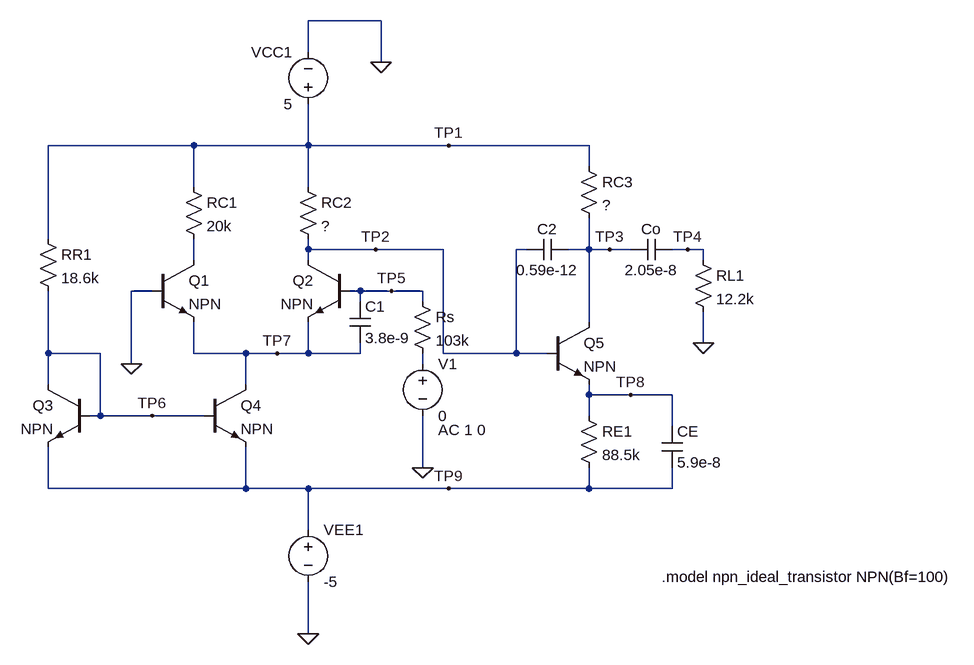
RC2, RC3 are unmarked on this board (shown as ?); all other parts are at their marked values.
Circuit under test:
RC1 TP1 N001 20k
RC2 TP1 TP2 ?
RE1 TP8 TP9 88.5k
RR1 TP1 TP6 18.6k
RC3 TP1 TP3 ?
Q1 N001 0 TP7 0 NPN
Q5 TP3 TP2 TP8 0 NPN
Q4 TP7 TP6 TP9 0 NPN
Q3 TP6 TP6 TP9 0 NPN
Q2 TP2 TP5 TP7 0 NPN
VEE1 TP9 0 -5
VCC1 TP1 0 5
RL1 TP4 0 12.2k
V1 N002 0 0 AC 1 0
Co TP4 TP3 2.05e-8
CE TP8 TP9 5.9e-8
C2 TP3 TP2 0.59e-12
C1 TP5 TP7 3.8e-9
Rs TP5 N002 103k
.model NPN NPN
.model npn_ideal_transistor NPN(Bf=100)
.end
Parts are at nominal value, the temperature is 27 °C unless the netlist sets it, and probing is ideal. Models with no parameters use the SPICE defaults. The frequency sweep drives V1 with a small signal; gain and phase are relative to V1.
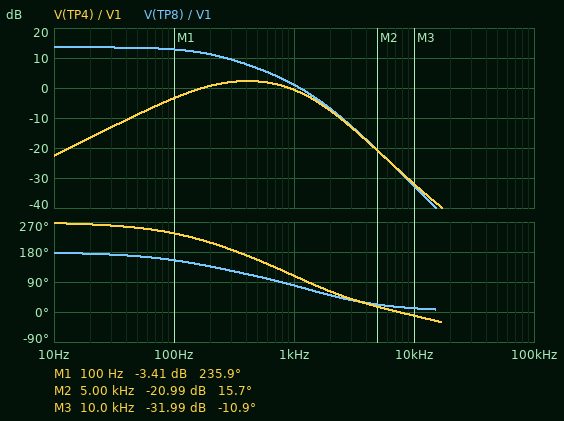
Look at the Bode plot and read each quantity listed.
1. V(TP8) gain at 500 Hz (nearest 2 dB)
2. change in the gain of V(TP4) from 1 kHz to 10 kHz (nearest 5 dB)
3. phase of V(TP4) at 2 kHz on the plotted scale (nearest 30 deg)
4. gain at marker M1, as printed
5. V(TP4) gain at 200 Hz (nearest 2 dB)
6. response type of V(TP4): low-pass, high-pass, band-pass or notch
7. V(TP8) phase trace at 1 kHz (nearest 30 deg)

6 dB
-30 dB
60 deg
-3.41 dB
0 dB
band-pass
90 deg
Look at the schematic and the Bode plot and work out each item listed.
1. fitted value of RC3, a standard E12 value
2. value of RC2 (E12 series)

47 kΩ
10 kΩ
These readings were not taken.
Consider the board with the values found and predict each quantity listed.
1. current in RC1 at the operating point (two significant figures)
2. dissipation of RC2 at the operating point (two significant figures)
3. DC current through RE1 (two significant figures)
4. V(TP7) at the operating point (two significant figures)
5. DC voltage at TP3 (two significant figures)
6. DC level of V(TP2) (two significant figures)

290 µA
120 µW
92 µA
-760 mV
3.2 V
3.9 V
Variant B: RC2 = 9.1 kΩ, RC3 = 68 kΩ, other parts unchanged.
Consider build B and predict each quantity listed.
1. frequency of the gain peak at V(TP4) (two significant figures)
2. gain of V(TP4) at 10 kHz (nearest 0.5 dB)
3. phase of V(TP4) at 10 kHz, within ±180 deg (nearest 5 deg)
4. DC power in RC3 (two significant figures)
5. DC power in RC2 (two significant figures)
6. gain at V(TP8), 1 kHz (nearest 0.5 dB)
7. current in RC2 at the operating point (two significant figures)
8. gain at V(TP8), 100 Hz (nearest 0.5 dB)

420 Hz
-32.5 dB
0 deg
49 µW
140 µW
1.0 dB
120 µA
12.5 dB
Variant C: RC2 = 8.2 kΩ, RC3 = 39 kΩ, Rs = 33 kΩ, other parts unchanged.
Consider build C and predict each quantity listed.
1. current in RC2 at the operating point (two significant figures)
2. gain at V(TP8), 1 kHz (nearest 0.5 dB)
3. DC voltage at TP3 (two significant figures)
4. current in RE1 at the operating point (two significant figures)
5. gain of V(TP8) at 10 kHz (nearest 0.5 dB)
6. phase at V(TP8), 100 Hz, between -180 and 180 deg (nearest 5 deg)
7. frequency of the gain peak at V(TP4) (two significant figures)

150 µA
9.5 dB
3.1 V
91 µA
-17.5 dB
160 deg
500 Hz
